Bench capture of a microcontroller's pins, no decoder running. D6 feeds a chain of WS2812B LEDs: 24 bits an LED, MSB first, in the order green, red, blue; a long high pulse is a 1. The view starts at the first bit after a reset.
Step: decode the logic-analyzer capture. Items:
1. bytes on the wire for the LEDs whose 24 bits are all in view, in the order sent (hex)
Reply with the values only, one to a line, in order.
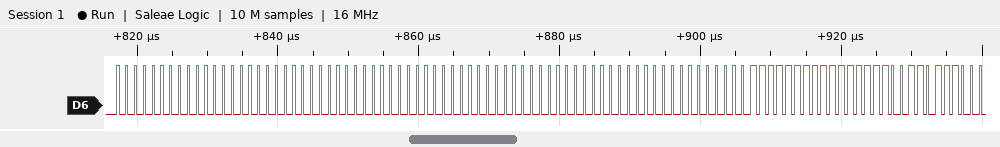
00 00 00 00 00 00 00 00 00 FF FF 37
